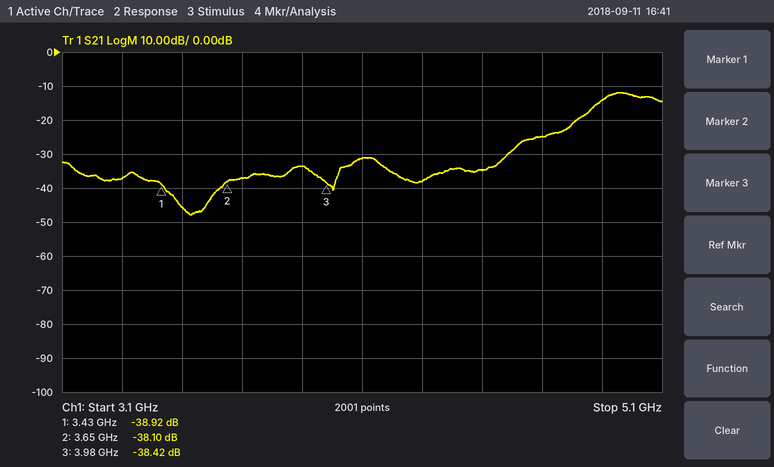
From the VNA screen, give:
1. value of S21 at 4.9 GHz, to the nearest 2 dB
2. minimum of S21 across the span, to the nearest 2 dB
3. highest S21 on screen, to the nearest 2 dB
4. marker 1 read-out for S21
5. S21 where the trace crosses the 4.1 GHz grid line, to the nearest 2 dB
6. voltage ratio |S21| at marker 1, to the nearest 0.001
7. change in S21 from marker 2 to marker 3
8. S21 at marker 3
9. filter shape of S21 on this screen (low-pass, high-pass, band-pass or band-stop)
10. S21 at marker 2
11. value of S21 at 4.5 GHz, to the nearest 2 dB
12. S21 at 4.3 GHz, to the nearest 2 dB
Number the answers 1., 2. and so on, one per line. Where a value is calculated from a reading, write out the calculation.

1. -14 dB
2. -48 dB
3. -12 dB
4. -38.92 dB
5. -32 dB
6. 10^(-38.92/20) ≈ 0.011
7. -38.42 − (-38.1) = -0.32 dB
8. -38.42 dB
9. high-pass
10. -38.10 dB
11. -34 dB
12. -38 dB
